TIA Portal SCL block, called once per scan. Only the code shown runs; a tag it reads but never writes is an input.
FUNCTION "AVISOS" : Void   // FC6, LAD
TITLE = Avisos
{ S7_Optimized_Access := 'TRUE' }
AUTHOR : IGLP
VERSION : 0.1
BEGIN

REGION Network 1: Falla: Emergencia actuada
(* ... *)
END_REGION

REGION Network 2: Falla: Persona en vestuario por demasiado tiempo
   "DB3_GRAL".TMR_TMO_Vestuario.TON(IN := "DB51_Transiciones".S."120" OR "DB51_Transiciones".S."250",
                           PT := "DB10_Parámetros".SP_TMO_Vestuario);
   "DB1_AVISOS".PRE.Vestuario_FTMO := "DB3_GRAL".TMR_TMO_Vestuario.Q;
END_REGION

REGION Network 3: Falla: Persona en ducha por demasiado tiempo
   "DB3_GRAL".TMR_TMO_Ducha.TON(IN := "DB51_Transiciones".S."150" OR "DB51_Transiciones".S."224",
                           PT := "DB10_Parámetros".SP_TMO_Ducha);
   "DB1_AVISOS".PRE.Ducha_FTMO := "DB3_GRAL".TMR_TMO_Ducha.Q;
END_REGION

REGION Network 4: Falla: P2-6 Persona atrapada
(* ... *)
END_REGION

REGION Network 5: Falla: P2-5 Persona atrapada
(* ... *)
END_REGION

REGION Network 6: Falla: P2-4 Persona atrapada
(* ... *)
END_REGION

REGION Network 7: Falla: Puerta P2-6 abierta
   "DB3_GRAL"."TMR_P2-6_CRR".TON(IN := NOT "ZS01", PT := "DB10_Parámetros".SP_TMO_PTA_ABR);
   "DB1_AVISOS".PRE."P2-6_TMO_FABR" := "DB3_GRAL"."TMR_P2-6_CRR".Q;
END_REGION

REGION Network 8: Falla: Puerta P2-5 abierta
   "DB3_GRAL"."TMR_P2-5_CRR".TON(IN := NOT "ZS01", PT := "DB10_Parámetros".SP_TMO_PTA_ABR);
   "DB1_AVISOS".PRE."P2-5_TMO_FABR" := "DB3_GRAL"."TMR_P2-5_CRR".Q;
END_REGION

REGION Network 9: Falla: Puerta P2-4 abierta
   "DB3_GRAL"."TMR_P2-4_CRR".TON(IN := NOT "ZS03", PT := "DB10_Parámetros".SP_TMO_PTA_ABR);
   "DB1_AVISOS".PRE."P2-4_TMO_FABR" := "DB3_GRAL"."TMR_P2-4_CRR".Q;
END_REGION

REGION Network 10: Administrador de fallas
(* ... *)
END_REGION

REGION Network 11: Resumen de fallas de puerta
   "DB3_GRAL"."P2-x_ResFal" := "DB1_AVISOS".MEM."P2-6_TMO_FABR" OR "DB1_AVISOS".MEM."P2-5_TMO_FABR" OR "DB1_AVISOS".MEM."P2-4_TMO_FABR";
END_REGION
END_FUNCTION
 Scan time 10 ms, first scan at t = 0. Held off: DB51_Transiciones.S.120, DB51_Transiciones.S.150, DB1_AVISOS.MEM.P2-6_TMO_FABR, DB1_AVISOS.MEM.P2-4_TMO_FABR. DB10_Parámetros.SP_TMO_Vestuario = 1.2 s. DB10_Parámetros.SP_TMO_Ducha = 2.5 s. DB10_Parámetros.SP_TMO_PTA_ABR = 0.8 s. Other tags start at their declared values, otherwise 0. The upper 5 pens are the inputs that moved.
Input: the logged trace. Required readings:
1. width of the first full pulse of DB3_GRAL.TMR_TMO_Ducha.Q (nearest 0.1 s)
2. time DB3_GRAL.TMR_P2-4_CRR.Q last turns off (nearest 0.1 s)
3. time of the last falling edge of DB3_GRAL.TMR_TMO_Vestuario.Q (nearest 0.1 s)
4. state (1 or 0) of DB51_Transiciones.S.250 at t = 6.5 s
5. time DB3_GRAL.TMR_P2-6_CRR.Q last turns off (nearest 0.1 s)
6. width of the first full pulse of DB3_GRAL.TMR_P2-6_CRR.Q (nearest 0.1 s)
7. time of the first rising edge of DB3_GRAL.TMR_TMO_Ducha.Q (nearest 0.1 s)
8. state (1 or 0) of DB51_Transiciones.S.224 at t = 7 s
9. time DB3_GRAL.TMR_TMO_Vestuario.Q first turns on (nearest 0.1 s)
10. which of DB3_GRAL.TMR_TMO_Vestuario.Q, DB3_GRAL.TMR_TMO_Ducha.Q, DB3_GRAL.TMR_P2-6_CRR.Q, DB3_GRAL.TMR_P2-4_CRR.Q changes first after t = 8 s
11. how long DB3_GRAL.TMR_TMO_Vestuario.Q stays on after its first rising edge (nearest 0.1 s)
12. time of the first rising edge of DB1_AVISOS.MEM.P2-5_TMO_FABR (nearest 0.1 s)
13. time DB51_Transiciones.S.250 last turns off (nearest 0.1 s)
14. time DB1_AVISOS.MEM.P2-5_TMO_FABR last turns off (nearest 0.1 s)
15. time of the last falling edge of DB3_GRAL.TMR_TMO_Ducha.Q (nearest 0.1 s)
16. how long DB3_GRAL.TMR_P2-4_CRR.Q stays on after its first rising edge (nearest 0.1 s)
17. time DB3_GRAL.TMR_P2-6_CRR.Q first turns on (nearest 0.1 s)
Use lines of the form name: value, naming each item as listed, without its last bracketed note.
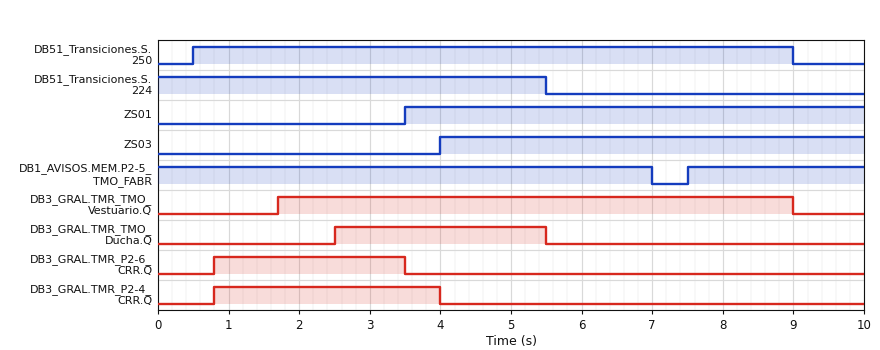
width of the first full pulse of DB3_GRAL.TMR_TMO_Ducha.Q: 3.0 s
time DB3_GRAL.TMR_P2-4_CRR.Q last turns off: 4.0 s
time of the last falling edge of DB3_GRAL.TMR_TMO_Vestuario.Q: 9.0 s
state (1 or 0) of DB51_Transiciones.S.250 at t = 6.5 s: 1
time DB3_GRAL.TMR_P2-6_CRR.Q last turns off: 3.5 s
width of the first full pulse of DB3_GRAL.TMR_P2-6_CRR.Q: 2.7 s
time of the first rising edge of DB3_GRAL.TMR_TMO_Ducha.Q: 2.5 s
state (1 or 0) of DB51_Transiciones.S.224 at t = 7 s: 0
time DB3_GRAL.TMR_TMO_Vestuario.Q first turns on: 1.7 s
which of DB3_GRAL.TMR_TMO_Vestuario.Q, DB3_GRAL.TMR_TMO_Ducha.Q, DB3_GRAL.TMR_P2-6_CRR.Q, DB3_GRAL.TMR_P2-4_CRR.Q changes first after t = 8 s: DB3_GRAL.TMR_TMO_Vestuario.Q
how long DB3_GRAL.TMR_TMO_Vestuario.Q stays on after its first rising edge: 7.3 s
time of the first rising edge of DB1_AVISOS.MEM.P2-5_TMO_FABR: 7.5 s
time DB51_Transiciones.S.250 last turns off: 9.0 s
time DB1_AVISOS.MEM.P2-5_TMO_FABR last turns off: 7.0 s
time of the last falling edge of DB3_GRAL.TMR_TMO_Ducha.Q: 5.5 s
how long DB3_GRAL.TMR_P2-4_CRR.Q stays on after its first rising edge: 3.2 s
time DB3_GRAL.TMR_P2-6_CRR.Q first turns on: 0.8 s
